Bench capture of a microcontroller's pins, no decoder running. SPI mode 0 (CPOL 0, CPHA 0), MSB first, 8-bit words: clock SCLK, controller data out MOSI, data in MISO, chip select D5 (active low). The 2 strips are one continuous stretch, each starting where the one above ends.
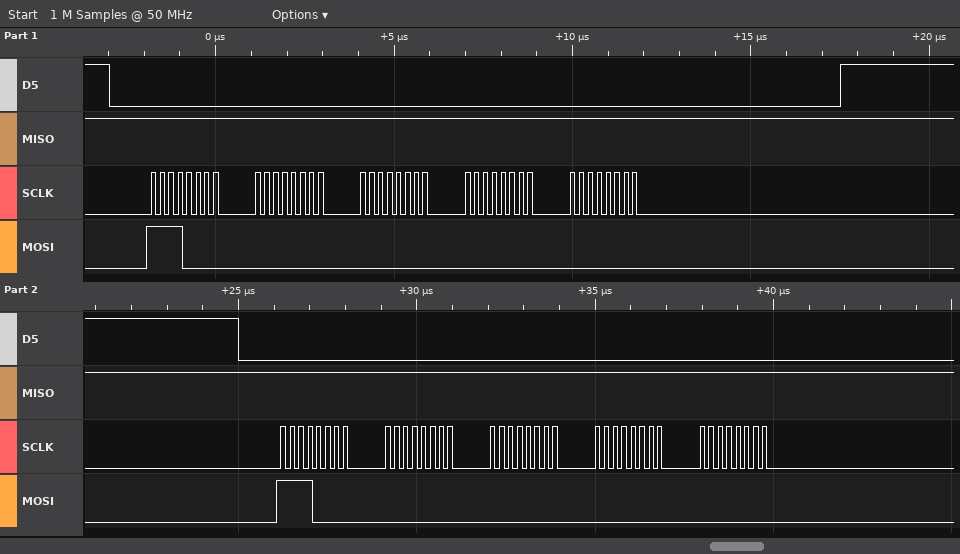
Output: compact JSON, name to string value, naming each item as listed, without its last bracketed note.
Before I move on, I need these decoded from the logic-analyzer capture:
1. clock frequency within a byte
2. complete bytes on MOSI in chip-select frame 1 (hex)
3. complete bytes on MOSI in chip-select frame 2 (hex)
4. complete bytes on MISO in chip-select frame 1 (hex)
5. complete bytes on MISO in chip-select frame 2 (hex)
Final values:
{"clock frequency within a byte": "4 MHz", "complete bytes on MOSI in chip-select frame 1": "F0 00 00 00 00", "complete bytes on MOSI in chip-select frame 2": "F0 00 00 00 00", "complete bytes on MISO in chip-select frame 1": "FF FF FF FF FF", "complete bytes on MISO in chip-select frame 2": "FF FF FF FF FF"}
